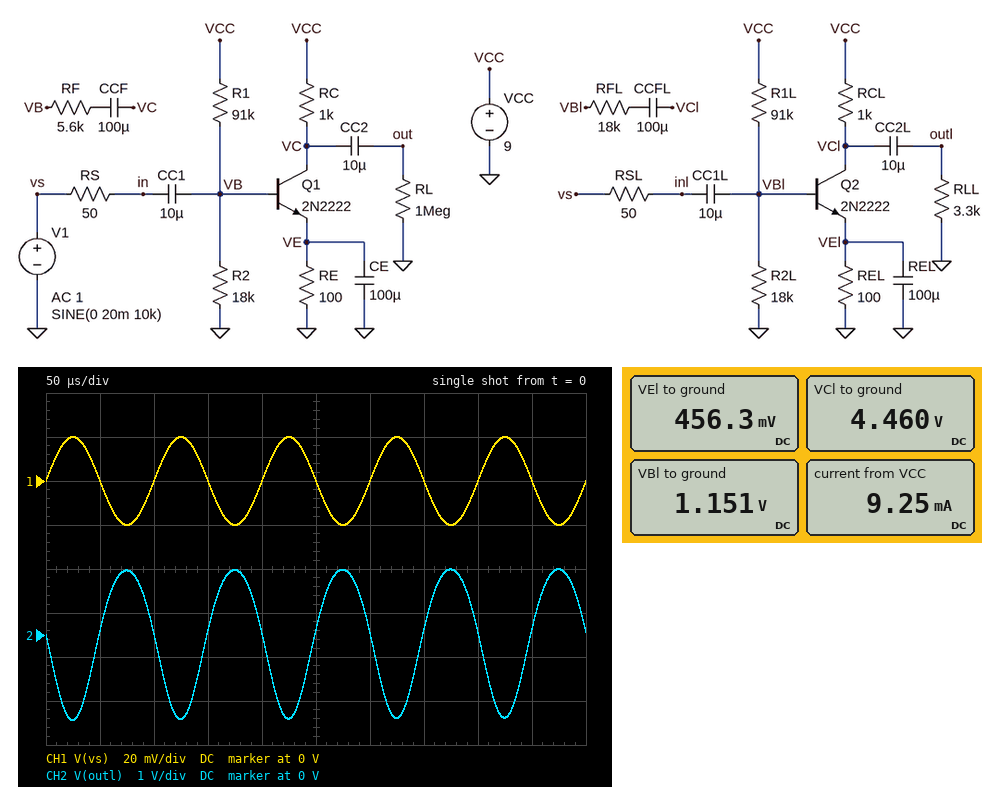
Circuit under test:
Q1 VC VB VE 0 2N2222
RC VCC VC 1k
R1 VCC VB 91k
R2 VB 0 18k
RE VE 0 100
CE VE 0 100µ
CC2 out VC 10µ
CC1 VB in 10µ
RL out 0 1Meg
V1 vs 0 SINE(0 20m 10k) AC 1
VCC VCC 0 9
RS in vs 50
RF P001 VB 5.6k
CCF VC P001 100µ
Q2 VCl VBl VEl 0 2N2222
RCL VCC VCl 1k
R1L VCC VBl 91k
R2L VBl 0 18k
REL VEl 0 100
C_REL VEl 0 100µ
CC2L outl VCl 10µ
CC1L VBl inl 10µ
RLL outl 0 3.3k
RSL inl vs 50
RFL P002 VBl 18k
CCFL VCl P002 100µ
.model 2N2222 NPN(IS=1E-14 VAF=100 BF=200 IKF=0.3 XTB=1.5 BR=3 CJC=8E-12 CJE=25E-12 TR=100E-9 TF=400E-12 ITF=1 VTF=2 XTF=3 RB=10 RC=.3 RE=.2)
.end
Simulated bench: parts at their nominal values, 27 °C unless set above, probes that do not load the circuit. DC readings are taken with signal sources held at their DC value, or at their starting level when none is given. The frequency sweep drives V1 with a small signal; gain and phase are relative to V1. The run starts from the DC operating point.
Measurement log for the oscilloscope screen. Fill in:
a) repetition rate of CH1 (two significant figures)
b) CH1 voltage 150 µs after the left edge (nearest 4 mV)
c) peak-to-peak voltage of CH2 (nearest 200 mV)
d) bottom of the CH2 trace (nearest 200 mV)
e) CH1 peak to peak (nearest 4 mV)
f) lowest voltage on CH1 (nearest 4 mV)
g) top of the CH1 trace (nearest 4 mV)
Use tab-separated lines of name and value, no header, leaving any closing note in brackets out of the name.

repetition rate of CH1	10 kHz
CH1 voltage 150 µs after the left edge	0 V
peak-to-peak voltage of CH2	3.4 V
bottom of the CH2 trace	-2.0 V
CH1 peak to peak	40 mV
lowest voltage on CH1	-20 mV
top of the CH1 trace	20 mV
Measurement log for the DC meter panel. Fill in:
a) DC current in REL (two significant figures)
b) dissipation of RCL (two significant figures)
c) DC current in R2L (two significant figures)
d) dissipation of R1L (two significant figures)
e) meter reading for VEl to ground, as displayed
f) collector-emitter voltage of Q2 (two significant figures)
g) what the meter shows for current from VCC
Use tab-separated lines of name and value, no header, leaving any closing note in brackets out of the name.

DC current in REL	4.6 mA
dissipation of RCL	21 mW
DC current in R2L	64 µA
dissipation of R1L	680 µW
meter reading for VEl to ground, as displayed	456.3 mV
collector-emitter voltage of Q2	4.0 V
what the meter shows for current from VCC	9.25 mA
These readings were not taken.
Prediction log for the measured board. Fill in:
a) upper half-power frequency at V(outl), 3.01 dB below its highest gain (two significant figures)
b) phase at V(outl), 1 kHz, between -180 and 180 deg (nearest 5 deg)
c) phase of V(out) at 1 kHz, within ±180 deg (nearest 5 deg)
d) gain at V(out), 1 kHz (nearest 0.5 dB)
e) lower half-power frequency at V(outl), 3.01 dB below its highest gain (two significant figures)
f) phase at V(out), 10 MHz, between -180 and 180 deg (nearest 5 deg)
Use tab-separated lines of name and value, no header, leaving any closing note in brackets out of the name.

upper half-power frequency at V(outl), 3.01 dB below its highest gain	5.2 MHz
phase at V(outl), 1 kHz, between -180 and 180 deg	-165 deg
phase of V(out) at 1 kHz, within ±180 deg	-165 deg
gain at V(out), 1 kHz	35.0 dB
lower half-power frequency at V(outl), 3.01 dB below its highest gain	280 Hz
phase at V(out), 10 MHz, between -180 and 180 deg	125 deg
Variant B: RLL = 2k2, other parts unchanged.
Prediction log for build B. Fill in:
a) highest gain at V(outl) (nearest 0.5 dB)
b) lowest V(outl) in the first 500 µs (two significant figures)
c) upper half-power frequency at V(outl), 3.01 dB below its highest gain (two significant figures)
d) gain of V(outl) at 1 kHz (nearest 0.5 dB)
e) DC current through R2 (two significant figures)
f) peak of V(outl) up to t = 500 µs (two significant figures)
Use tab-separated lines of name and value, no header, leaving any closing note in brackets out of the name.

highest gain at V(outl)	38.0 dB
lowest V(outl) in the first 500 µs	-1.8 V
upper half-power frequency at V(outl), 3.01 dB below its highest gain	5.6 MHz
gain of V(outl) at 1 kHz	37.5 dB
DC current through R2	64 µA
peak of V(outl) up to t = 500 µs	1.4 V
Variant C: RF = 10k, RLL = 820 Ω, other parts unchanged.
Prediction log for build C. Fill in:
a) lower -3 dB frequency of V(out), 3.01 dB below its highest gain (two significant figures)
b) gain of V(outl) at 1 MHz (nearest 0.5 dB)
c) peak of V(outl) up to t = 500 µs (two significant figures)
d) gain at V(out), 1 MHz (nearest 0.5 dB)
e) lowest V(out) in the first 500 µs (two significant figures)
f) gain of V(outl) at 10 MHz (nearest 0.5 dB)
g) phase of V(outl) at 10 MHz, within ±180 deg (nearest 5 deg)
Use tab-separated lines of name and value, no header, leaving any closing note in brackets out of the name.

lower -3 dB frequency of V(out), 3.01 dB below its highest gain	290 Hz
gain of V(outl) at 1 MHz	35.0 dB
peak of V(outl) up to t = 500 µs	970 mV
gain at V(out), 1 MHz	38.0 dB
lowest V(out) in the first 500 µs	-1.7 V
gain of V(outl) at 10 MHz	30.5 dB
phase of V(outl) at 10 MHz, within ±180 deg	125 deg
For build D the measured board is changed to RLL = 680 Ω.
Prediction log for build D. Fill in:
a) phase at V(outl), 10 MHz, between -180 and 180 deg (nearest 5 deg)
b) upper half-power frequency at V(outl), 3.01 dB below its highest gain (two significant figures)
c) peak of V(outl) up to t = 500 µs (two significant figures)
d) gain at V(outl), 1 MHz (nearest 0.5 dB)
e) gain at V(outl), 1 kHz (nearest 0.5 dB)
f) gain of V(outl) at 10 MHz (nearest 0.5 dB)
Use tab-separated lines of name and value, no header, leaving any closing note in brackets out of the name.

phase at V(outl), 10 MHz, between -180 and 180 deg	125 deg
upper half-power frequency at V(outl), 3.01 dB below its highest gain	7.6 MHz
peak of V(outl) up to t = 500 µs	880 mV
gain at V(outl), 1 MHz	34.5 dB
gain at V(outl), 1 kHz	34.0 dB
gain of V(outl) at 10 MHz	30.0 dB
